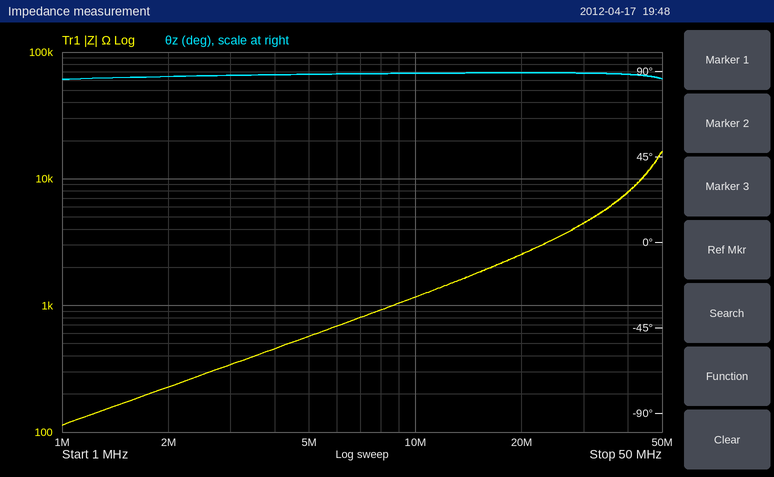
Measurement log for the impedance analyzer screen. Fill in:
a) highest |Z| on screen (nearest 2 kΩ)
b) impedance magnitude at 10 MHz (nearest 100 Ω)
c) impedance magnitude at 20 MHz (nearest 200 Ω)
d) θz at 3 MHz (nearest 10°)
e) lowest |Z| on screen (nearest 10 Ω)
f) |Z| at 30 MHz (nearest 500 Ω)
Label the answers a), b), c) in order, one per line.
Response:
a) 16 kΩ
b) 1.2 kΩ
c) 2.6 kΩ
d) 90°
e) 110 Ω
f) 4.5 kΩ
